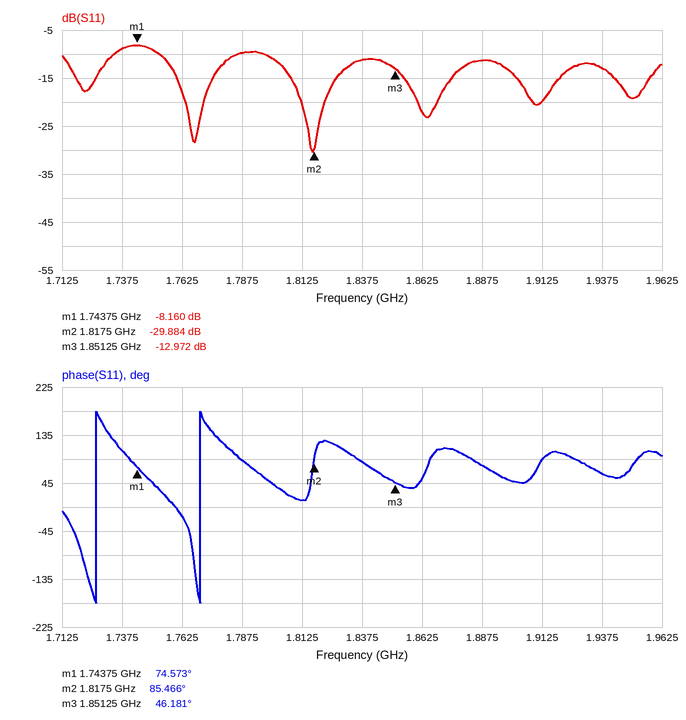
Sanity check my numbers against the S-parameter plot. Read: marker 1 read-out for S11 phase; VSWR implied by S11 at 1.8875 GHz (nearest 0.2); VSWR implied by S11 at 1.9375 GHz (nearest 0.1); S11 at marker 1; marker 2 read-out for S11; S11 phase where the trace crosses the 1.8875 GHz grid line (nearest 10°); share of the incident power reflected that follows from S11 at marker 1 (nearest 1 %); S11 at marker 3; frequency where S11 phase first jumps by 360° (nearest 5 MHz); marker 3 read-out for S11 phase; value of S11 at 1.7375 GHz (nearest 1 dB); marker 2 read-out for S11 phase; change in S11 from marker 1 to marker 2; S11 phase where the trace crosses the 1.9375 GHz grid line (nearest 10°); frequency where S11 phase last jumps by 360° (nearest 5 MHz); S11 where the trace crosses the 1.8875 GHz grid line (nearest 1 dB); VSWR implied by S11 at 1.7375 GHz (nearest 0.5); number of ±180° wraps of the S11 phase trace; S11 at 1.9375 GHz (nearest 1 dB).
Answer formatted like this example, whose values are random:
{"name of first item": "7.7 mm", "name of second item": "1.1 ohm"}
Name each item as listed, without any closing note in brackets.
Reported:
{"marker 1 read-out for S11 phase": "74.573°", "VSWR implied by S11 at 1.8875 GHz": "1.8", "VSWR implied by S11 at 1.9375 GHz": "1.6", "S11 at marker 1": "-8.160 dB", "marker 2 read-out for S11": "-29.884 dB", "S11 phase where the trace crosses the 1.8875 GHz grid line": "80°", "share of the incident power reflected that follows from S11 at marker 1": "15 %", "S11 at marker 3": "-12.972 dB", "frequency where S11 phase first jumps by 360°": "1.725 GHz", "marker 3 read-out for S11 phase": "46.181°", "value of S11 at 1.7375 GHz": "-9 dB", "marker 2 read-out for S11 phase": "85.466°", "change in S11 from marker 1 to marker 2": "-21.724 dB", "S11 phase where the trace crosses the 1.9375 GHz grid line": "60°", "frequency where S11 phase last jumps by 360°": "1.770 GHz", "S11 where the trace crosses the 1.8875 GHz grid line": "-11 dB", "VSWR implied by S11 at 1.7375 GHz": "2.0", "number of ±180° wraps of the S11 phase trace": "2", "S11 at 1.9375 GHz": "-13 dB"}
